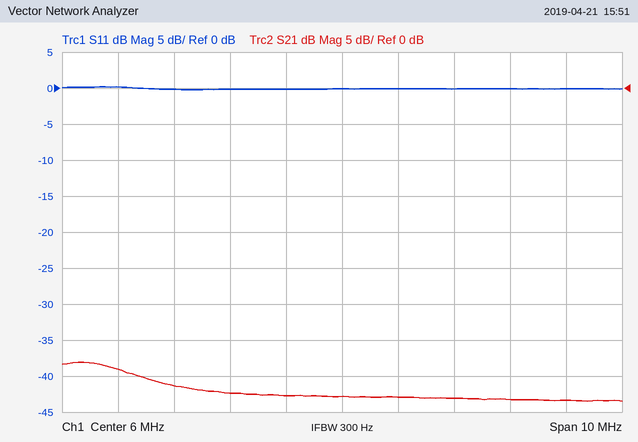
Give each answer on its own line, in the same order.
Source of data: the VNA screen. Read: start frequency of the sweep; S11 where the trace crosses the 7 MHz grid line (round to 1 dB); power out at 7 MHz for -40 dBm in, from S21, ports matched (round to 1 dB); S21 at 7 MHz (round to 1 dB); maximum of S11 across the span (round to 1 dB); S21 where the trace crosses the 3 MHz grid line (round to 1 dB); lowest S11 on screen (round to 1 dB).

1 MHz
0 dB
-83 dBm
-43 dB
0 dB
-41 dB
0 dB
